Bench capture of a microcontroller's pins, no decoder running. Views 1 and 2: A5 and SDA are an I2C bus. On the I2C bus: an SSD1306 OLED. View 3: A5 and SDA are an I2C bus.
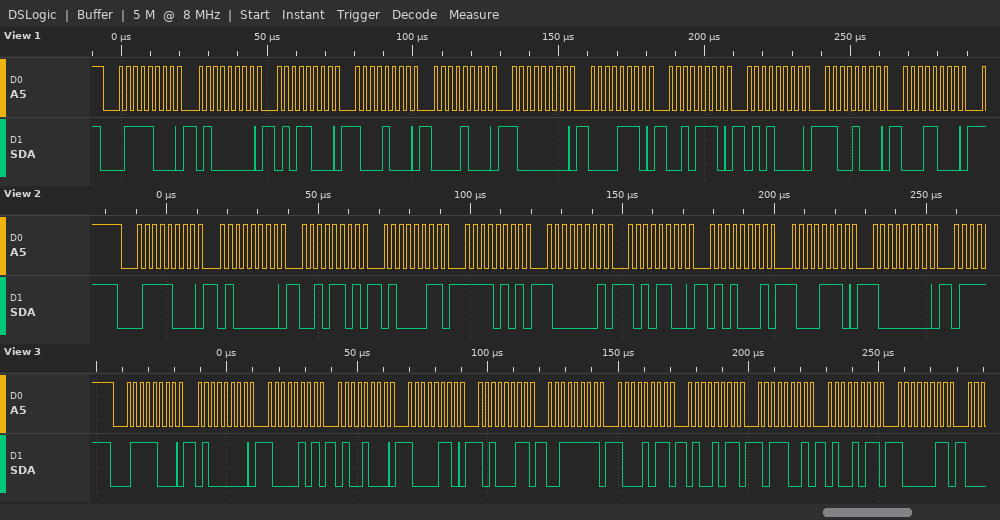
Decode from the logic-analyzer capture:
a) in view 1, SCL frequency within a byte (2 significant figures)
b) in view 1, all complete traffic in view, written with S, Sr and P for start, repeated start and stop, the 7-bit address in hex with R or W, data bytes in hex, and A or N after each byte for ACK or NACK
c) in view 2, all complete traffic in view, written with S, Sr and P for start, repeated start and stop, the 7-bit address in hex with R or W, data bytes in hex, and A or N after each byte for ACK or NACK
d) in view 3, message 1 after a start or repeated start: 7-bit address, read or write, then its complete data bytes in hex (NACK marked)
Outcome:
400 kHz
S 3CW A 40 A 58 A 88 A 08 A 80 A 0E A 2E A 50 A C8 A 18 A
S 3CW A 40 A 2D A 43 A F5 A 81 A AC A 51 A 8E A 80 A
0x3C write: 40 85 48 86 A3 3F 8B 4B B9 4B 83
